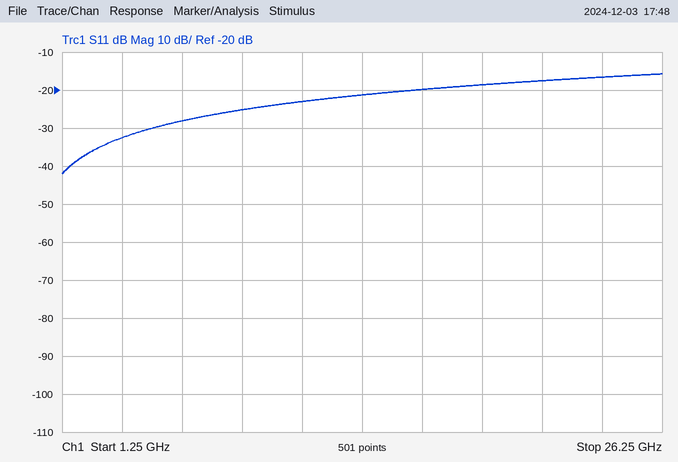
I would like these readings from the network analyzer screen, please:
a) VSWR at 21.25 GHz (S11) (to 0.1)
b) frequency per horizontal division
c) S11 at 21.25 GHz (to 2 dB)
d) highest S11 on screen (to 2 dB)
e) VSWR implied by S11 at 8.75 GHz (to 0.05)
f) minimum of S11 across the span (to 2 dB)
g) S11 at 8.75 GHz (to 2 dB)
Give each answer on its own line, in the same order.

1.3
2.5 GHz
-18 dB
-16 dB
1.10
-42 dB
-26 dB
